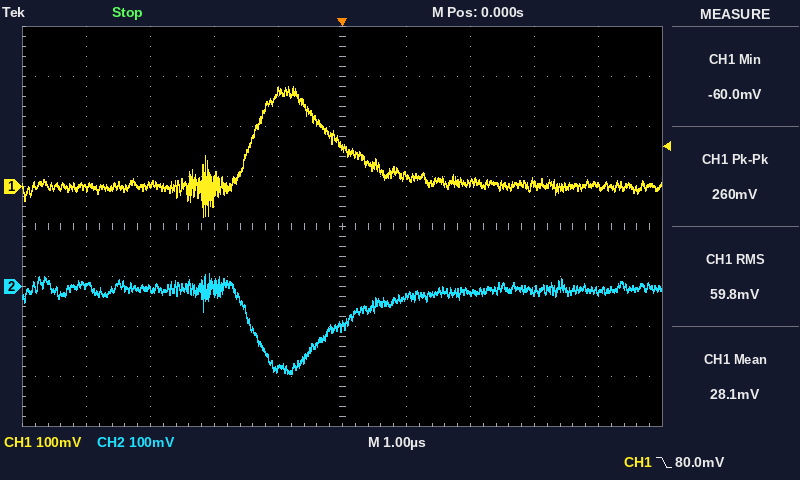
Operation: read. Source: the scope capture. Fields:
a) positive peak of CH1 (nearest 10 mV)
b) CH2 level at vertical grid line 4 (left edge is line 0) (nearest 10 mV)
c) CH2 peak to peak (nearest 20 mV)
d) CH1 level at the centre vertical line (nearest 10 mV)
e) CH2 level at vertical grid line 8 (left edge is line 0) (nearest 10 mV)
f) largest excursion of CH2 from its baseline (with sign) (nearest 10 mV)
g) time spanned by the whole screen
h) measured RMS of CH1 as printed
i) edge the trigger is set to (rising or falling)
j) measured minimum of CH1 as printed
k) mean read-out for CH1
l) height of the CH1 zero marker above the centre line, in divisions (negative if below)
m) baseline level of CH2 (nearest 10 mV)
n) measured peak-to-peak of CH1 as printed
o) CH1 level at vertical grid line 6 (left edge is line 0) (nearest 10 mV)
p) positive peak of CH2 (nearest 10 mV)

200 mV
-160 mV
200 mV
80 mV
-10 mV
-170 mV
10 µs
59.8 mV
falling
-60.0 mV
28.1 mV
+0.8 div
-10 mV
260 mV
20 mV
30 mV
